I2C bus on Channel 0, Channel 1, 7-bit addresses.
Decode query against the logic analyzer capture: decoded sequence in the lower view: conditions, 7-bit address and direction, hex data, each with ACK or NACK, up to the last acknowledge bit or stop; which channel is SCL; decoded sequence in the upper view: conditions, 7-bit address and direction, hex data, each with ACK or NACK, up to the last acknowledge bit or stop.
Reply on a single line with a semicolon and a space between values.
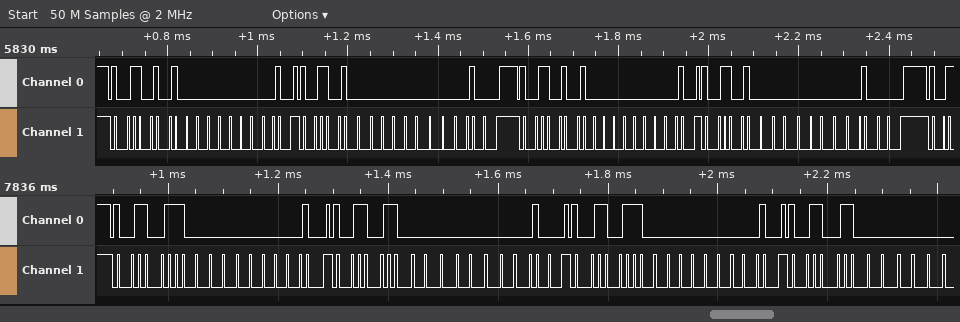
start, address 5B read ACK, 00 NACK, stop, start, address 5B write ACK, 01 ACK, stop, start, address 5B read ACK, 00 NACK, stop, start, address 5B write ACK; Channel 1; start, address 5A read ACK, 00 NACK, stop, start, address 5A write ACK, 01 ACK, stop, start, address 5A read ACK, 00 NACK, stop, start, address 5A write ACK, 02 ACK, stop
